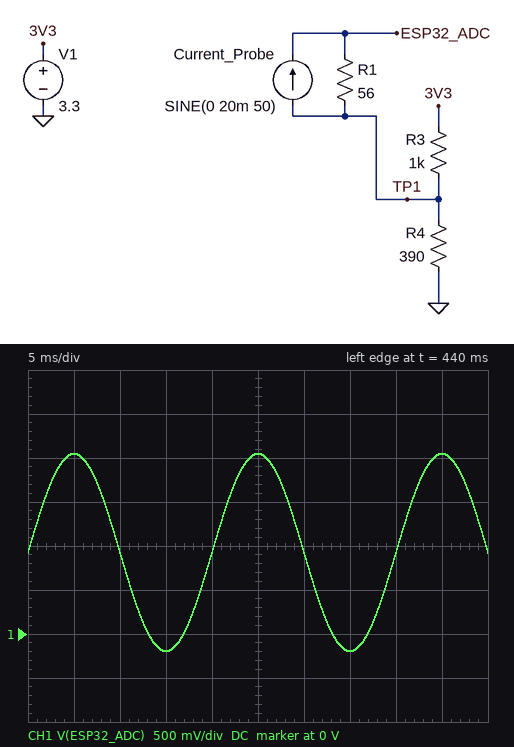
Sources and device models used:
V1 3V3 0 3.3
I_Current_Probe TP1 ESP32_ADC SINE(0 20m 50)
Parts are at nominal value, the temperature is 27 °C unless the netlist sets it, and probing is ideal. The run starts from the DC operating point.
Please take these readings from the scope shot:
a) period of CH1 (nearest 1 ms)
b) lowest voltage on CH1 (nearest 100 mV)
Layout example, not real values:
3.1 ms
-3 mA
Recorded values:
20 ms
-200 mV
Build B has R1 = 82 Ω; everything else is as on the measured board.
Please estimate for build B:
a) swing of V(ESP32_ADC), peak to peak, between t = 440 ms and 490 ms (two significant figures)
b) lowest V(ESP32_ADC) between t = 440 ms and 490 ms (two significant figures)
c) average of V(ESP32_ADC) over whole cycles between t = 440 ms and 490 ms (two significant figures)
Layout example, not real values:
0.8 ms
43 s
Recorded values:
3.3 V
-710 mV
930 mV
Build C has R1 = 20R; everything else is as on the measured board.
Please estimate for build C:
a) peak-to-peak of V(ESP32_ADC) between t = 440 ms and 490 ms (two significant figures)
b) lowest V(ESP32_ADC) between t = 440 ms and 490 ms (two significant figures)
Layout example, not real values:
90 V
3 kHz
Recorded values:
800 mV
530 mV
